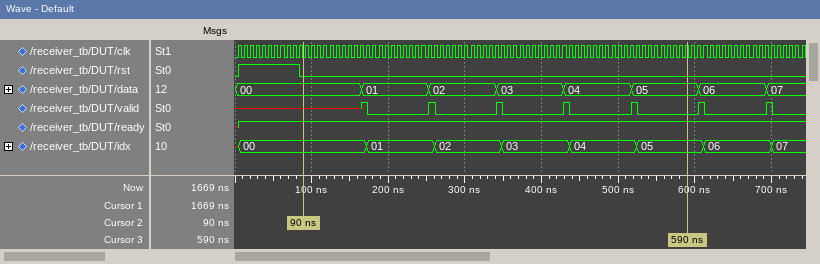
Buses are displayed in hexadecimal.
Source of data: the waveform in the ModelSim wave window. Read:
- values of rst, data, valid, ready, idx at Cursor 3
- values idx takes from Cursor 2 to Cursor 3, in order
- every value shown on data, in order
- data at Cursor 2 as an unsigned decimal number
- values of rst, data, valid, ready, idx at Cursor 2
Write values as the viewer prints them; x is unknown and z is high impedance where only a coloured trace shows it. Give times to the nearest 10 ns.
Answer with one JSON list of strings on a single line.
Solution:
["rst=0, data=05, valid=0, ready=1, idx=05", "00, 01, 02, 03, 04, 05", "00, 01, 02, 03, 04, 05, 06, 07", "0", "rst=0, data=00, valid=x, ready=1, idx=00"]
